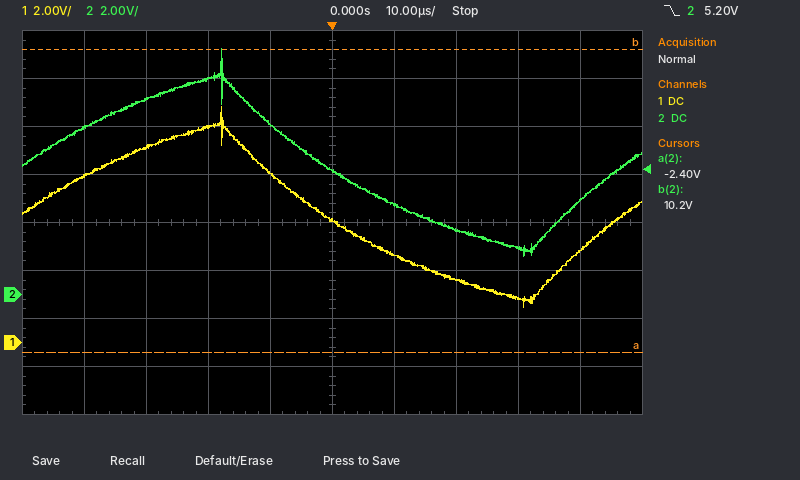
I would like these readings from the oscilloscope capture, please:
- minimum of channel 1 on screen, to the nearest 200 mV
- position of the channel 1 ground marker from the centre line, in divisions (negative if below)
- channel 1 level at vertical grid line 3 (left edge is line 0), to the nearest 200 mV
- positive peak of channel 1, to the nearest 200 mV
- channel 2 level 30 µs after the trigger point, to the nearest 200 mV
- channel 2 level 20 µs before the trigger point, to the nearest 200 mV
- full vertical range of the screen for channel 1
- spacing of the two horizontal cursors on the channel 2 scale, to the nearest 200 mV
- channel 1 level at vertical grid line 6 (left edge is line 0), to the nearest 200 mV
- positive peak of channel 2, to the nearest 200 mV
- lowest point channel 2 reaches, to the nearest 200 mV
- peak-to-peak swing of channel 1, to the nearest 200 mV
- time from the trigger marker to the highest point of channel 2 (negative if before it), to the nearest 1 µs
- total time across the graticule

1.4 V
-2.5 div
9.0 V
9.8 V
2.0 V
9.0 V
16 V
12.6 V
3.6 V
10.2 V
1.6 V
8.4 V
-18 µs
100 µs
